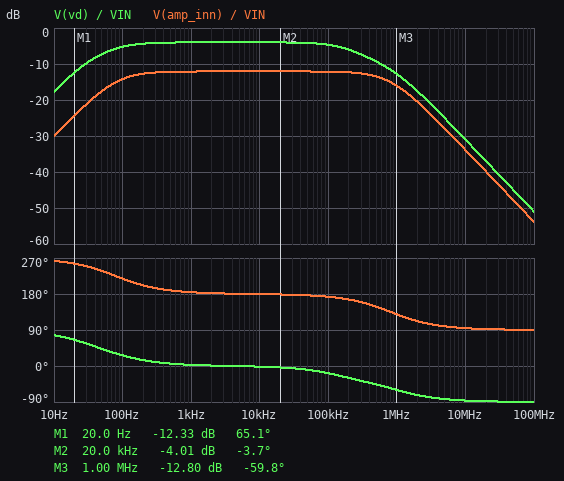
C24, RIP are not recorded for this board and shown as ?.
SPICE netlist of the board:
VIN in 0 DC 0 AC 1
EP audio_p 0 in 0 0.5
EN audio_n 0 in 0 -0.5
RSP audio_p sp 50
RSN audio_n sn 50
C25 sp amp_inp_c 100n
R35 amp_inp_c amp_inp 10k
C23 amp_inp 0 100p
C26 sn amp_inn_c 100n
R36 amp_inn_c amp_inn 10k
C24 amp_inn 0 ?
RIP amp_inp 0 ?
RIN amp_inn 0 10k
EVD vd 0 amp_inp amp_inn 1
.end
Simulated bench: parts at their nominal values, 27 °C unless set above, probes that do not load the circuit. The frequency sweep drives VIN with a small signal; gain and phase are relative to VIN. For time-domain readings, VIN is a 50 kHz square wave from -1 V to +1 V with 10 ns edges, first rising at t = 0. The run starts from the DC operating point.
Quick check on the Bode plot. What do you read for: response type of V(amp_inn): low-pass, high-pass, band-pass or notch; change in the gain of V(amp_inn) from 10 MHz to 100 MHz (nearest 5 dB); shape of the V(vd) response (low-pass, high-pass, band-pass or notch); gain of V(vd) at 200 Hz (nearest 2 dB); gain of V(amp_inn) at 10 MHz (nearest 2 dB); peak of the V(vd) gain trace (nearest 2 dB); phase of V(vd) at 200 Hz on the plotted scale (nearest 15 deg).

band-pass
-20 dB
band-pass
-4 dB
-34 dB
-4 dB
15 deg
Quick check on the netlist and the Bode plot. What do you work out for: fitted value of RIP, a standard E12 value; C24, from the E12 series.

33 kΩ
39 pF
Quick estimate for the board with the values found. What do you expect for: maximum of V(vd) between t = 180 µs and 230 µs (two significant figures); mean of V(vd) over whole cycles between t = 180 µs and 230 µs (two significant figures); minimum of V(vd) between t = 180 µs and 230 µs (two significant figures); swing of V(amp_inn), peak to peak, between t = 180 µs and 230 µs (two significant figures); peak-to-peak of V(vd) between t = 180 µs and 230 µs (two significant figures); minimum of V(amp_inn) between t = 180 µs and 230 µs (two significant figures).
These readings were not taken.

1.2 V
590 mV
-45 mV
500 mV
1.3 V
-480 mV
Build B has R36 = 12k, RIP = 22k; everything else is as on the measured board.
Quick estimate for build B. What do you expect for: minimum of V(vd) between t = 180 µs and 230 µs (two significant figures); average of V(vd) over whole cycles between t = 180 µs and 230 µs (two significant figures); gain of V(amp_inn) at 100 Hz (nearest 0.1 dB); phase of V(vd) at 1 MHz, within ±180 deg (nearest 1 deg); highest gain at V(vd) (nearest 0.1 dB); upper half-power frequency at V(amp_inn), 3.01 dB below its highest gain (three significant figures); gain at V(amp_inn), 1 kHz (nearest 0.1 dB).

-44 mV
530 mV
-14.7 dB
-62 deg
-4.9 dB
747 kHz
-12.9 dB
